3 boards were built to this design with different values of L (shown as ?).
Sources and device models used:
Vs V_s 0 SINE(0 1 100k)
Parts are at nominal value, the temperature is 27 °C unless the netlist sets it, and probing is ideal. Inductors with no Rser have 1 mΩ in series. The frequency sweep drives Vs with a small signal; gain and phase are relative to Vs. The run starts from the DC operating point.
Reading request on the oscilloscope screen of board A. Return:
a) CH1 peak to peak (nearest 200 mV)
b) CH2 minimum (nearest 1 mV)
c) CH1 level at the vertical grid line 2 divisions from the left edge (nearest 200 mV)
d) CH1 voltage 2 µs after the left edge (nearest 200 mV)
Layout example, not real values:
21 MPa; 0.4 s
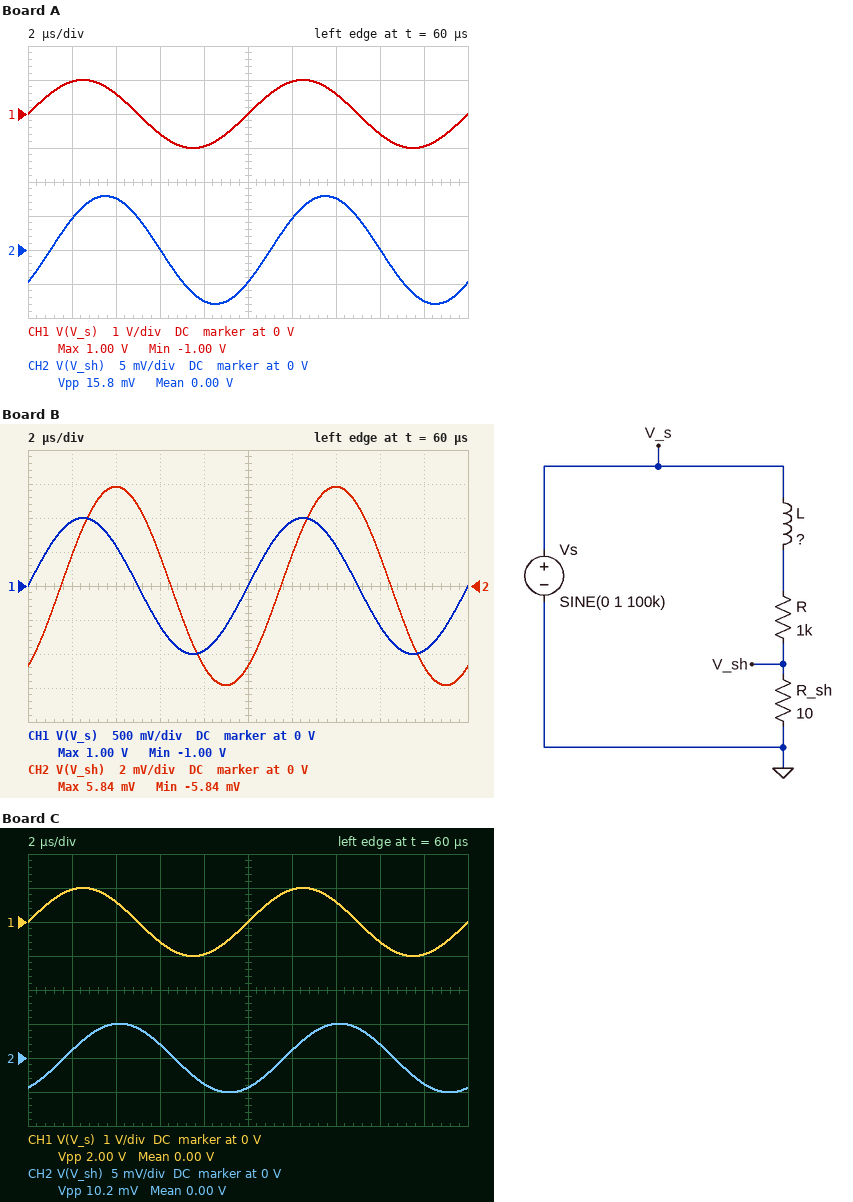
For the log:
2.0 V; -8 mV; 600 mV; 1.0 V
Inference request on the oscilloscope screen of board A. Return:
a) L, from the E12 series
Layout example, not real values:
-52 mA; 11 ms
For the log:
1.2 mH
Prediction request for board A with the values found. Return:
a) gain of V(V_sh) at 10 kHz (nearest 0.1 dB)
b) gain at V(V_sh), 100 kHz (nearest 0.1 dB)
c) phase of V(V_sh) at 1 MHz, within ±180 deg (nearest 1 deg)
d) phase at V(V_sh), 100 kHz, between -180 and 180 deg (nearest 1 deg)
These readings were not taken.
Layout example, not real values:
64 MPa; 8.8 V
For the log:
-40.1 dB; -42.0 dB; -82 deg; -37 deg
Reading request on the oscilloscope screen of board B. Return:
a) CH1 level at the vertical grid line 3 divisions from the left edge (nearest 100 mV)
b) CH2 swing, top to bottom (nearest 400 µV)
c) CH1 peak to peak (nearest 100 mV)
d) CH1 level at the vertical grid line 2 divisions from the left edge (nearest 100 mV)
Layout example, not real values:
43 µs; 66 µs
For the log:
-600 mV; 11.6 mV; 2.0 V; 600 mV
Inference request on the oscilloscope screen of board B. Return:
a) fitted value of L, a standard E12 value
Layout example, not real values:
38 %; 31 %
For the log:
2.2 mH
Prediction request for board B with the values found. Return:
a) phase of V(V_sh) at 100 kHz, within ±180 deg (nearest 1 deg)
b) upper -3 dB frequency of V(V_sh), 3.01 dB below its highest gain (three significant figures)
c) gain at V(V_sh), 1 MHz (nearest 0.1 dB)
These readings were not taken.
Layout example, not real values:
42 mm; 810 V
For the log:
-54 deg; 73.1 kHz; -62.8 dB
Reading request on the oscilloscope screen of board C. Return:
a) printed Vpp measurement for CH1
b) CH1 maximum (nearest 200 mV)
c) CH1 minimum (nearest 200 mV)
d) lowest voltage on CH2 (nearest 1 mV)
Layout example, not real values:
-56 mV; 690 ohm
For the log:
2.00 V; 1.0 V; -1.0 V; -5 mV
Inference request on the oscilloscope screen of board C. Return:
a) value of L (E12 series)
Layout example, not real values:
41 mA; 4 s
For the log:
2.7 mH
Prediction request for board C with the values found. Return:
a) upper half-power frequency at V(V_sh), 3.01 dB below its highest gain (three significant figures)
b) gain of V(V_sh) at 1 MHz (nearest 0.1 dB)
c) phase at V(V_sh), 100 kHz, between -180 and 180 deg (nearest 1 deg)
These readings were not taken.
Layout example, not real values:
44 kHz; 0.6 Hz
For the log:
59.5 kHz; -64.6 dB; -59 deg
